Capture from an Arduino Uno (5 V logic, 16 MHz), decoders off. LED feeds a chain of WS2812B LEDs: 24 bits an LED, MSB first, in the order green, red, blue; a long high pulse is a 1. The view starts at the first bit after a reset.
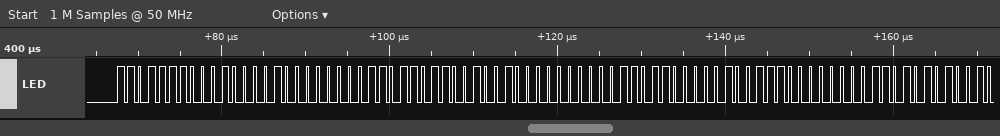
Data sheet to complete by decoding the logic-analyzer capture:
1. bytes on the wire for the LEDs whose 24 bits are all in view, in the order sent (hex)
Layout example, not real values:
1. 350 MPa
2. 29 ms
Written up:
1. DE 21 00 DB 24 00 D8 27 00
